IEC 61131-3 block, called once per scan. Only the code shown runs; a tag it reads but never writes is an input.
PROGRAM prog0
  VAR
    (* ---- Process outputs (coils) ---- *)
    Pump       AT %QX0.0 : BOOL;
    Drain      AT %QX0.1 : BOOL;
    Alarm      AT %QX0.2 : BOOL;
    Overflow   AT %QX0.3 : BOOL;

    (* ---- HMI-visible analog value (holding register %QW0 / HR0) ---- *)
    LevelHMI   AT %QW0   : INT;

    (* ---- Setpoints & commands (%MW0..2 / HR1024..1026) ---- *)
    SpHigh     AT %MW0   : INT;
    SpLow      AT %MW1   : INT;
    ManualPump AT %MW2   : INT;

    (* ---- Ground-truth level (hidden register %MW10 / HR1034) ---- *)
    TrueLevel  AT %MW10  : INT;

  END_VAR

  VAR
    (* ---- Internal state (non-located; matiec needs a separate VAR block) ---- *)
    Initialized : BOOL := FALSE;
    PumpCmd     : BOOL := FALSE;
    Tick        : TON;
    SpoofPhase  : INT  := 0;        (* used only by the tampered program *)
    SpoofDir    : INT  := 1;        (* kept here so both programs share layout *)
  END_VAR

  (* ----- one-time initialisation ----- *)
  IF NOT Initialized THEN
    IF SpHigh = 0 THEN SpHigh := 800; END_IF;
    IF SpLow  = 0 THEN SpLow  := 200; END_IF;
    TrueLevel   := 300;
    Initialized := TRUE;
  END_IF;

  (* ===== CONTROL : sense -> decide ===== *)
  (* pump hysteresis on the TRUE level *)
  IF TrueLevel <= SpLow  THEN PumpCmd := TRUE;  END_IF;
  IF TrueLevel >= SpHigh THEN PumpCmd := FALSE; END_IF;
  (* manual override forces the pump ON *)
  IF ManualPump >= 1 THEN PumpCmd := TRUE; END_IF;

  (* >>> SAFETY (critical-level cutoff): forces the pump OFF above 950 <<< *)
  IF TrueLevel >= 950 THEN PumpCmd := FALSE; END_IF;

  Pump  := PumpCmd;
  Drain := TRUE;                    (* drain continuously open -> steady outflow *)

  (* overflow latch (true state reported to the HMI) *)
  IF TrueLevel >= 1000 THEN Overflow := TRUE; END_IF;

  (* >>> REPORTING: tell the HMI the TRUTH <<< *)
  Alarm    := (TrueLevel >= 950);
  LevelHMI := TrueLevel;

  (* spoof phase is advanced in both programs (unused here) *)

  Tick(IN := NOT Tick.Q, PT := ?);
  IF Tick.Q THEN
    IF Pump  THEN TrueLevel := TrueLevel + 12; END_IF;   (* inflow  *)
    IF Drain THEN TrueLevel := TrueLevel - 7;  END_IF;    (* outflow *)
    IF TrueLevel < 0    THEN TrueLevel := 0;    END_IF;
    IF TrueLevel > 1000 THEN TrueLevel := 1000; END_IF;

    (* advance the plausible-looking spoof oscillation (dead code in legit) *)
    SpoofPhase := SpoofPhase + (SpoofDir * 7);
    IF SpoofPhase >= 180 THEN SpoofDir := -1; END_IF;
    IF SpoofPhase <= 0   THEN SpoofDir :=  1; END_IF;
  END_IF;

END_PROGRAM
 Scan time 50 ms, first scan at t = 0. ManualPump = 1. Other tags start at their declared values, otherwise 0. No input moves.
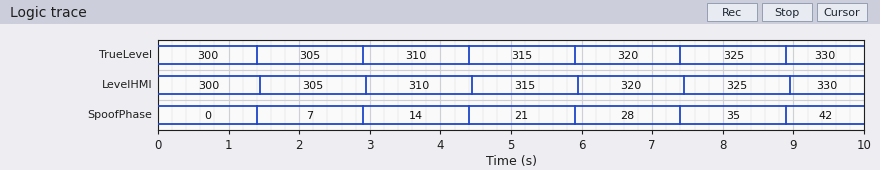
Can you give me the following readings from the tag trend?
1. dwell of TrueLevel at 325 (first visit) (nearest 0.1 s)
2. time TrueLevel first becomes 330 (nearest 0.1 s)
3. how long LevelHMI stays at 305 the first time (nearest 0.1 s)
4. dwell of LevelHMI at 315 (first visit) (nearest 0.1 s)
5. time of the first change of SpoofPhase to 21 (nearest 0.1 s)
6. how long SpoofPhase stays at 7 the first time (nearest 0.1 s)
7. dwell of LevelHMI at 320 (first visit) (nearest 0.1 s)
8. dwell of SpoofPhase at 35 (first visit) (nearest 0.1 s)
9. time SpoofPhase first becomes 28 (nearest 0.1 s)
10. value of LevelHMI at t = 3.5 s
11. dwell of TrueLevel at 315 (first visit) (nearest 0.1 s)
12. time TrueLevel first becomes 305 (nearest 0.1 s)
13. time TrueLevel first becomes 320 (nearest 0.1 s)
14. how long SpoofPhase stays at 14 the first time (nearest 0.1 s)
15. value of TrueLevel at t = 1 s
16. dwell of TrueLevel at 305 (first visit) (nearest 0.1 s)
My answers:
1.5 s
8.9 s
1.5 s
1.5 s
4.4 s
1.5 s
1.5 s
1.5 s
5.9 s
310
1.5 s
1.4 s
5.9 s
1.5 s
300
1.5 s
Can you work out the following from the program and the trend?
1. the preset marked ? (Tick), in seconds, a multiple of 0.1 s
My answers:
1.4 s
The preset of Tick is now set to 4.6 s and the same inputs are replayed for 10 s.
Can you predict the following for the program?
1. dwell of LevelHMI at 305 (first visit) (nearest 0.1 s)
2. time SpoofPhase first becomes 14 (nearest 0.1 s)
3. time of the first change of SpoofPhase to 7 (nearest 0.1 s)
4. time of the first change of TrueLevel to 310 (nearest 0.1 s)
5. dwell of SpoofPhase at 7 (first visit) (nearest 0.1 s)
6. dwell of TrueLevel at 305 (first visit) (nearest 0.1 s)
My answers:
4.7 s
9.3 s
4.6 s
9.3 s
4.7 s
4.7 s
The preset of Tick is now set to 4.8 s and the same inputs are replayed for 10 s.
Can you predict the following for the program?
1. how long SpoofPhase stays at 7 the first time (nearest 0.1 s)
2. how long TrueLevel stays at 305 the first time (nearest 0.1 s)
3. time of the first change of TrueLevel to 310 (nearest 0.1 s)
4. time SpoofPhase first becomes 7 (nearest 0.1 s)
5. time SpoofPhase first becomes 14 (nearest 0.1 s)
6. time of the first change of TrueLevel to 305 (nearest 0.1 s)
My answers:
4.9 s
4.9 s
9.7 s
4.8 s
9.7 s
4.8 s
